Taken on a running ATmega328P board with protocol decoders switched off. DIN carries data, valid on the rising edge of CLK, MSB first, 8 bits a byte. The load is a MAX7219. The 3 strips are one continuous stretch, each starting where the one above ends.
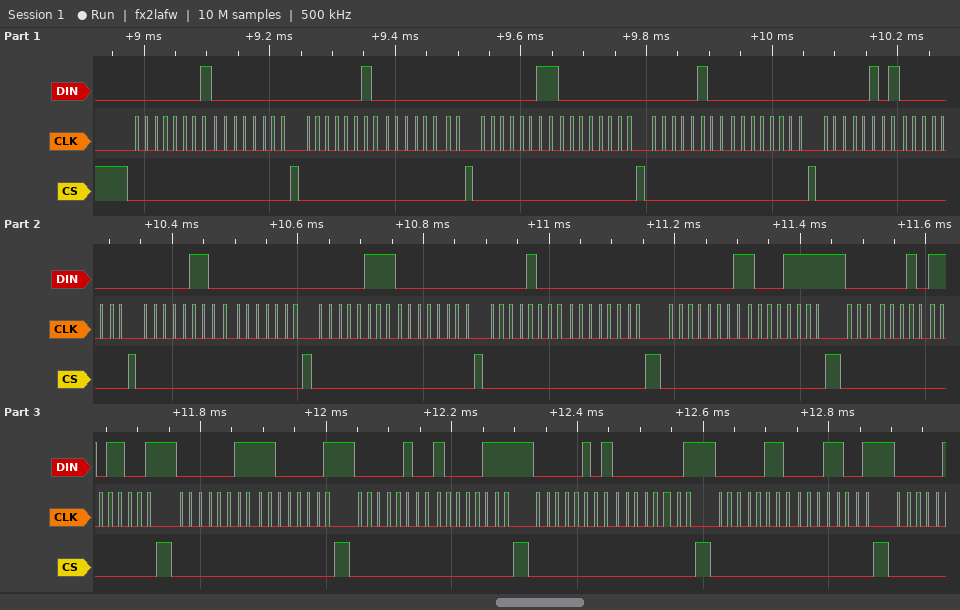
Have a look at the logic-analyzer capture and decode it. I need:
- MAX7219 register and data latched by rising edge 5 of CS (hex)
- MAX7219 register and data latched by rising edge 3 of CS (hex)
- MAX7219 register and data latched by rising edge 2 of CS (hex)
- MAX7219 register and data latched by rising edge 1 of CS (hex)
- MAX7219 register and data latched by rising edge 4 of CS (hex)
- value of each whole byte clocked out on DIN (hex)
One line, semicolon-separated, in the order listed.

register 0x5, data 0x00; register 0x3, data 0x00; register 0x2, data 0x00; register 0x1, data 0x00; register 0x4, data 0x00; 01 00 02 00 03 00 04 00 05 00 06 00 07 00 08 00 01 8F 02 D9 03 C1 04 87 05 01 06 19
